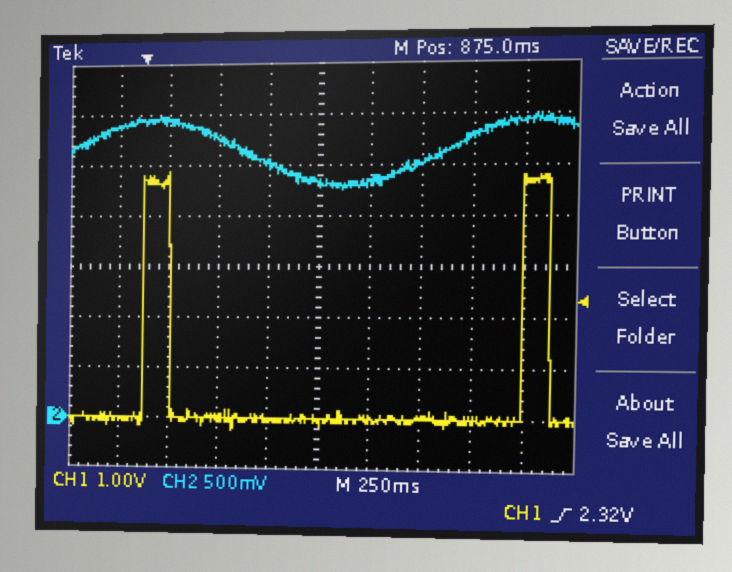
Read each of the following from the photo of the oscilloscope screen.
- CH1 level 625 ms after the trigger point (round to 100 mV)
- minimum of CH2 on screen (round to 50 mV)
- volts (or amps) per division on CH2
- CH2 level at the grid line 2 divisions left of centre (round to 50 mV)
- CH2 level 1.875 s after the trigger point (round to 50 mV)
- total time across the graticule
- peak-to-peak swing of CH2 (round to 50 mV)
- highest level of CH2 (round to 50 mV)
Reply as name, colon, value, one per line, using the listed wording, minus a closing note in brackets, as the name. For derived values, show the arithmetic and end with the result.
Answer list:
CH1 level 625 ms after the trigger point: 0.0 V
minimum of CH2 on screen: 2.25 V
volts (or amps) per division on CH2: 500 mV
CH2 level at the grid line 2 divisions left of centre: 2.80 V
CH2 level 1.875 s after the trigger point: 2.95 V
total time across the graticule: 2.5 s
peak-to-peak swing of CH2: 3.00 V − (2.25 V) = 750 mV
highest level of CH2: 3.00 V
